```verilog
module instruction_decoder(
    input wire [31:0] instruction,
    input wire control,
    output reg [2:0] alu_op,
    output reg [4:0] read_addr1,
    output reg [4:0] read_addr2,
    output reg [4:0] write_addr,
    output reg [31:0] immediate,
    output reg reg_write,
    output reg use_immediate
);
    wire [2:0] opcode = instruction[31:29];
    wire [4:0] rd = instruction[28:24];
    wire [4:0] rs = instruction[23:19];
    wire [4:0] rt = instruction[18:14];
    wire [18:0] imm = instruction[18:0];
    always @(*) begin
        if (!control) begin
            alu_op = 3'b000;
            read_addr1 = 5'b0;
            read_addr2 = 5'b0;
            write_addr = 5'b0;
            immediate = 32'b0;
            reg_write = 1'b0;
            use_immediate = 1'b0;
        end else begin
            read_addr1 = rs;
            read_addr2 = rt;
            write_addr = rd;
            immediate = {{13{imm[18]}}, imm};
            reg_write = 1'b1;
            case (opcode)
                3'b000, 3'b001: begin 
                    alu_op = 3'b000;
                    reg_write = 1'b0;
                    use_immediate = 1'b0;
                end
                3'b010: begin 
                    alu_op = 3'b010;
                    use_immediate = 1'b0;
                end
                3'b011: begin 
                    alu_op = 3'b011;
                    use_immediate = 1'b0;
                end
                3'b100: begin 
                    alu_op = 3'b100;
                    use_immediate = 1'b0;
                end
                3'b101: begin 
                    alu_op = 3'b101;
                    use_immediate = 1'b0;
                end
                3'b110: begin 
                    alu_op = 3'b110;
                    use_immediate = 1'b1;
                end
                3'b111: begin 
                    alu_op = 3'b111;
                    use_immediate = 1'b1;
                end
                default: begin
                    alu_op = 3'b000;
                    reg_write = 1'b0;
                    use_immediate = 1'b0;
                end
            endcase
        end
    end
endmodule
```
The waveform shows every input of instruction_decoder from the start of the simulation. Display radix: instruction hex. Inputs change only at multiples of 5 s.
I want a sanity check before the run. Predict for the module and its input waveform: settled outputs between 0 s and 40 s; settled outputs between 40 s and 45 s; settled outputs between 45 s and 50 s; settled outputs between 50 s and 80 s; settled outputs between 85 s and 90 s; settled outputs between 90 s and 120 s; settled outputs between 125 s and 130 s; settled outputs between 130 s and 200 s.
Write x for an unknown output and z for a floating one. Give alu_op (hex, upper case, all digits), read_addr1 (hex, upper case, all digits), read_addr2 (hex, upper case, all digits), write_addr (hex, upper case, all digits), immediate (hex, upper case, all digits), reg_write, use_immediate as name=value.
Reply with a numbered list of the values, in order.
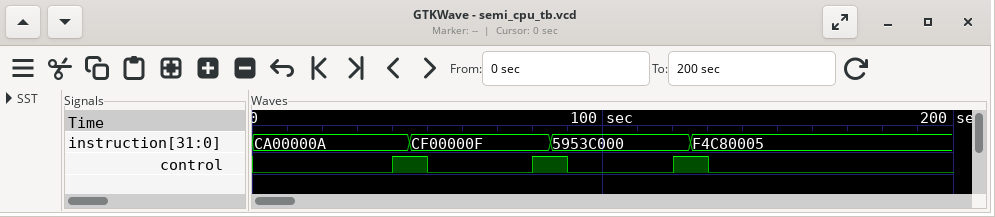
1. alu_op=0, read_addr1=00, read_addr2=00, write_addr=00, immediate=00000000, reg_write=0, use_immediate=0
2. alu_op=6, read_addr1=00, read_addr2=00, write_addr=0A, immediate=0000000A, reg_write=1, use_immediate=1
3. alu_op=6, read_addr1=00, read_addr2=00, write_addr=0F, immediate=0000000F, reg_write=1, use_immediate=1
4. alu_op=0, read_addr1=00, read_addr2=00, write_addr=00, immediate=00000000, reg_write=0, use_immediate=0
5. alu_op=2, read_addr1=0A, read_addr2=0F, write_addr=19, immediate=0003C000, reg_write=1, use_immediate=0
6. alu_op=0, read_addr1=00, read_addr2=00, write_addr=00, immediate=00000000, reg_write=0, use_immediate=0
7. alu_op=7, read_addr1=19, read_addr2=00, write_addr=14, immediate=00000005, reg_write=1, use_immediate=1
8. alu_op=0, read_addr1=00, read_addr2=00, write_addr=00, immediate=00000000, reg_write=0, use_immediate=0
